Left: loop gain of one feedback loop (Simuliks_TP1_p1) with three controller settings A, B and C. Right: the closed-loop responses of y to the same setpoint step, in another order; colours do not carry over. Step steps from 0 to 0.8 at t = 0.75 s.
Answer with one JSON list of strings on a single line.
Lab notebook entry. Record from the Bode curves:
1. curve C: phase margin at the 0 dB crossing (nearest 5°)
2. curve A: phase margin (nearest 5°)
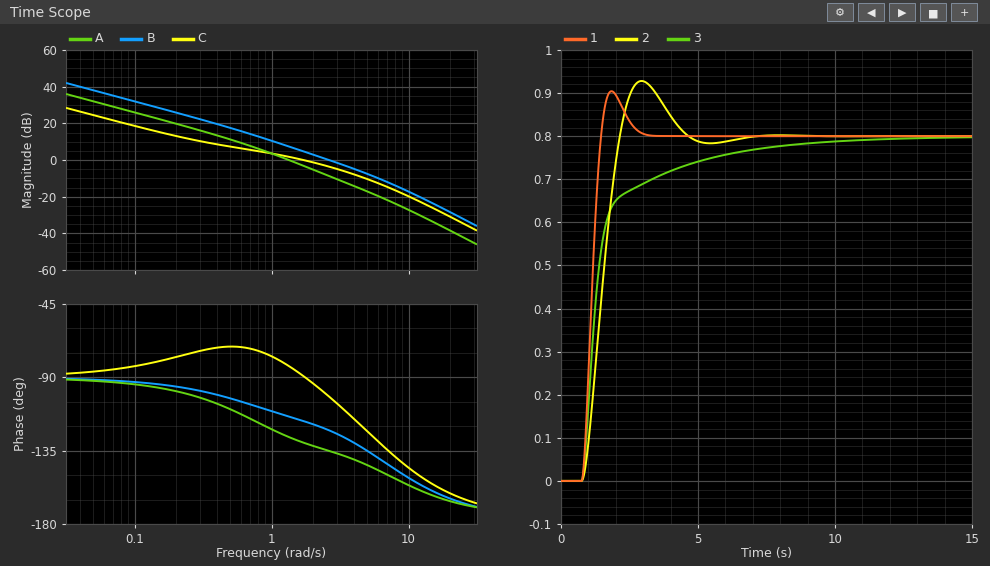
["90°", "55°"]
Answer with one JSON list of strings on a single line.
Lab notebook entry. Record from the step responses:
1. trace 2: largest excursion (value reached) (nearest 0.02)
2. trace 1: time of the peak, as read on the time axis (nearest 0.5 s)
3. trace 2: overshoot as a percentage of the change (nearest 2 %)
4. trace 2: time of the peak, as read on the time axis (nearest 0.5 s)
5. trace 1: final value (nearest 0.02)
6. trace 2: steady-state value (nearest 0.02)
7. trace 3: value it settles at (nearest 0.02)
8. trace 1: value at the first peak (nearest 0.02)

["0.92", "2.0 s", "16 %", "3.0 s", "0.80", "0.80", "0.80", "0.90"]
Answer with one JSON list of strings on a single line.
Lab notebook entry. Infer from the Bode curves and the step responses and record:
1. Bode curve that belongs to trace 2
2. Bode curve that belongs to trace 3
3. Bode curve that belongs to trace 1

["A", "C", "B"]
